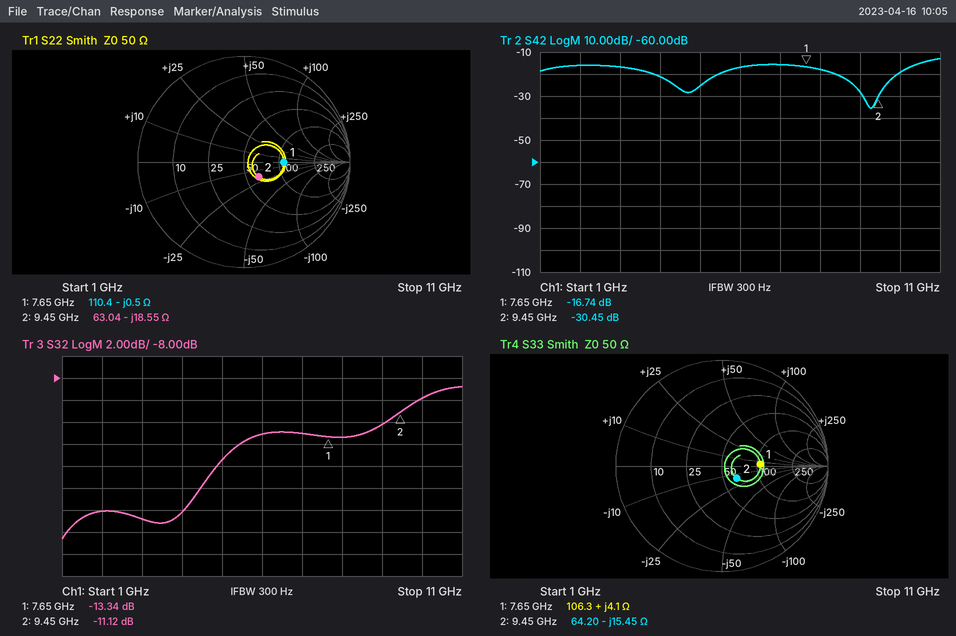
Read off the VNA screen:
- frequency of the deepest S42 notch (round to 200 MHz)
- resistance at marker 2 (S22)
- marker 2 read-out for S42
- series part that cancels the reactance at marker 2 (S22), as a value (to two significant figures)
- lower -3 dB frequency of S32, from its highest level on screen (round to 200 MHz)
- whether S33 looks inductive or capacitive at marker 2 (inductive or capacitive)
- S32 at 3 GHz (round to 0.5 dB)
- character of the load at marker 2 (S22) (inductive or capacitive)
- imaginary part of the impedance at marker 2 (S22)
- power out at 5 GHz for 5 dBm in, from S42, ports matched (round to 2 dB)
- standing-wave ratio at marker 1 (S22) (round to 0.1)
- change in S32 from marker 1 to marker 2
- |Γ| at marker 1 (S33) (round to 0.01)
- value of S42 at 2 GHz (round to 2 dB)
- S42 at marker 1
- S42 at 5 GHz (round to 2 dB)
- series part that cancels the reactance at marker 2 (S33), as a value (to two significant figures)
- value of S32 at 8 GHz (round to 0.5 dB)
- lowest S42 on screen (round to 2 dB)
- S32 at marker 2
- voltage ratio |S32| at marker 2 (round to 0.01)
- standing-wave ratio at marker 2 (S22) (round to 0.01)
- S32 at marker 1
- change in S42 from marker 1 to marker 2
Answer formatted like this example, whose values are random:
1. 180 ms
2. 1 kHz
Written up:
1. 9.2 GHz
2. 63.04 Ω
3. -30.45 dB
4. 310 pH
5. 9.2 GHz
6. capacitive
7. -21.0 dB
8. capacitive
9. -18.55 Ω
10. -20 dBm
11. 2.2
12. 2.22 dB
13. 0.36
14. -16 dB
15. -16.74 dB
16. -26 dB
17. 260 pH
18. -13.5 dB
19. -36 dB
20. -11.12 dB
21. 0.28
22. 1.49
23. -13.34 dB
24. -13.71 dB
